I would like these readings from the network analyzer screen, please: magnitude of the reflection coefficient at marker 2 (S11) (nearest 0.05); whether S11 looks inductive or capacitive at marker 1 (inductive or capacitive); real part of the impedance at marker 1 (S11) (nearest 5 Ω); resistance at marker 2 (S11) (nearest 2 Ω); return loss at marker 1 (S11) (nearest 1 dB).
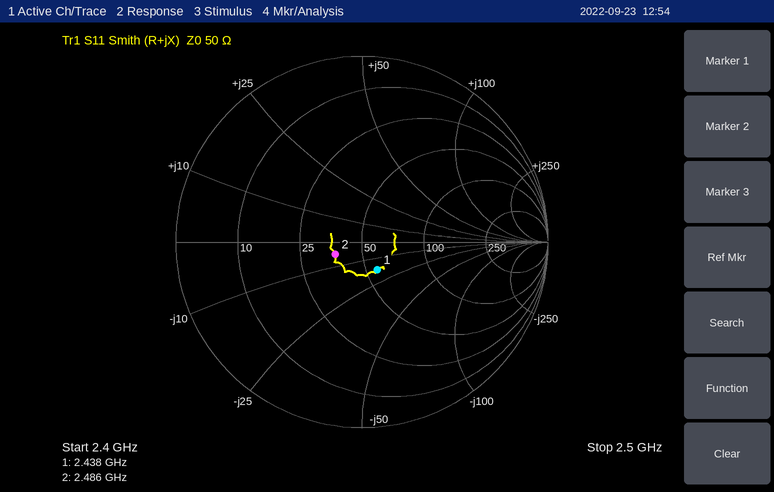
0.15
capacitive
55 Ω
38 Ω
15 dB
